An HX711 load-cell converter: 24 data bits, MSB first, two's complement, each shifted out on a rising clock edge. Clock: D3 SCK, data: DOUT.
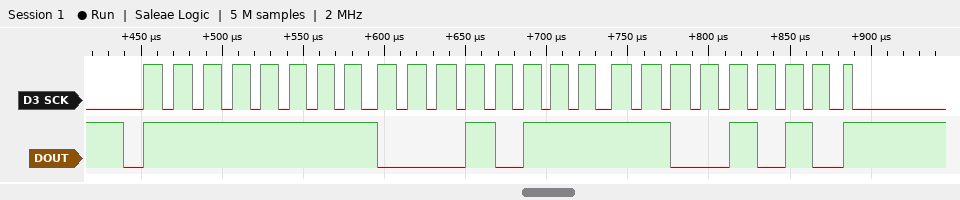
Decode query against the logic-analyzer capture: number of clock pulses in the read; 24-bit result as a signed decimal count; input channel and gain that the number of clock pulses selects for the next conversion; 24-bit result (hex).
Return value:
25
-59446
channel A, gain 128
0xFF17CA
